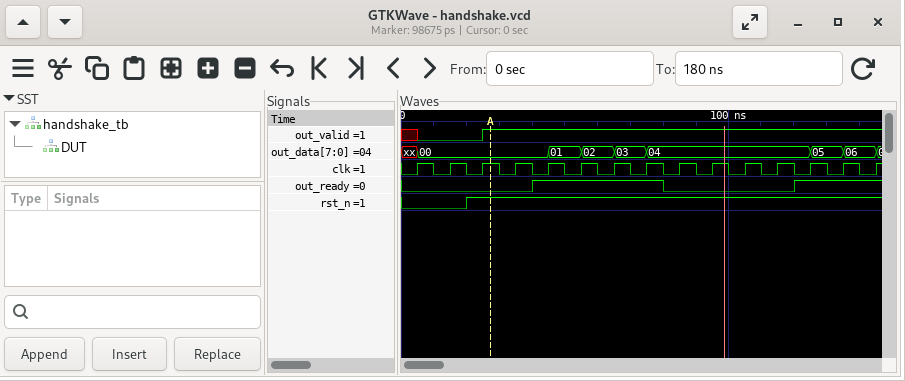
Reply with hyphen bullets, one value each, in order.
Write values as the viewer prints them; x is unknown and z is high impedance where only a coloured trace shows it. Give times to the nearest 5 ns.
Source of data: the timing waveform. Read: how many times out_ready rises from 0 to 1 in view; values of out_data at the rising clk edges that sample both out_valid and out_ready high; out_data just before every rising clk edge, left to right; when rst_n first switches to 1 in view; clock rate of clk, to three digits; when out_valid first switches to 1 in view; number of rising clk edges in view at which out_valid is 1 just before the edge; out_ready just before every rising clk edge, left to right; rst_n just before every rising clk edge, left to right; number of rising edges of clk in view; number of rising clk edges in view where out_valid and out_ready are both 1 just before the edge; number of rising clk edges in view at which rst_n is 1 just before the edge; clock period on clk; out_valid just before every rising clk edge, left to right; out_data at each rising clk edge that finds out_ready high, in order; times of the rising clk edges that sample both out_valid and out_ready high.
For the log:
- 2
- 00, 01, 02, 03, 04, 05, 06
- xx, 00, 00, 00, 00, 01, 02, 03, 04, 04, 04, 04, 04, 05, 06
- 20 ns
- 100 MHz
- 25 ns
- 12
- 0 0 0 0 1 1 1 1 0 0 0 0 1 1 1
- 0 0 1 1 1 1 1 1 1 1 1 1 1 1 1
- 15
- 7
- 13
- 10 ns
- x 0 0 1 1 1 1 1 1 1 1 1 1 1 1
- 00, 01, 02, 03, 04, 05, 06
- 45 ns, 55 ns, 65 ns, 75 ns, 125 ns, 135 ns, 145 ns
